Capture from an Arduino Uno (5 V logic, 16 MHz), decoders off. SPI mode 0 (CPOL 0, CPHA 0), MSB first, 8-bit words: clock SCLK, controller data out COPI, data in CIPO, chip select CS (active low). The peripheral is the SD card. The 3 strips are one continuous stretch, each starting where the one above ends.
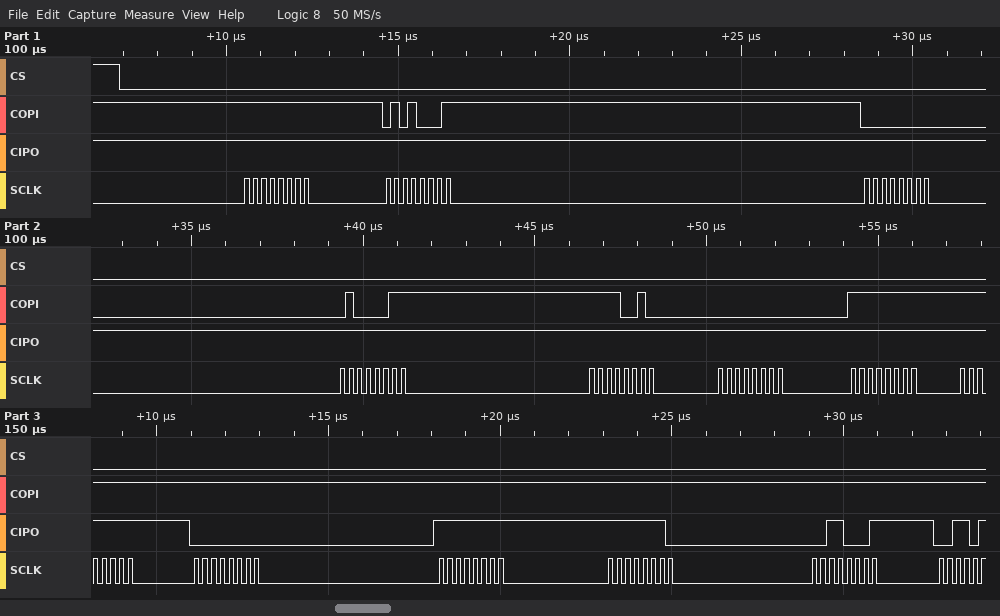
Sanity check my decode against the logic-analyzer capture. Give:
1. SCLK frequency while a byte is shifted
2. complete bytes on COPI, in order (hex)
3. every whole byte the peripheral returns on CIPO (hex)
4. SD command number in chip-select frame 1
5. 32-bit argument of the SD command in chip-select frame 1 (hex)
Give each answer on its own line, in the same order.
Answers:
4 MHz
FF 51 00 43 F2 00 FF FF FF FF FF FF
FF FF FF FF FF FF FF FF 00 FF FE 31
CMD17
0x0043F200
